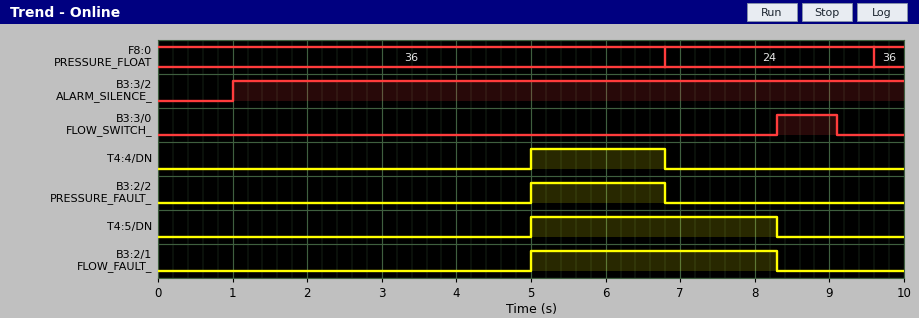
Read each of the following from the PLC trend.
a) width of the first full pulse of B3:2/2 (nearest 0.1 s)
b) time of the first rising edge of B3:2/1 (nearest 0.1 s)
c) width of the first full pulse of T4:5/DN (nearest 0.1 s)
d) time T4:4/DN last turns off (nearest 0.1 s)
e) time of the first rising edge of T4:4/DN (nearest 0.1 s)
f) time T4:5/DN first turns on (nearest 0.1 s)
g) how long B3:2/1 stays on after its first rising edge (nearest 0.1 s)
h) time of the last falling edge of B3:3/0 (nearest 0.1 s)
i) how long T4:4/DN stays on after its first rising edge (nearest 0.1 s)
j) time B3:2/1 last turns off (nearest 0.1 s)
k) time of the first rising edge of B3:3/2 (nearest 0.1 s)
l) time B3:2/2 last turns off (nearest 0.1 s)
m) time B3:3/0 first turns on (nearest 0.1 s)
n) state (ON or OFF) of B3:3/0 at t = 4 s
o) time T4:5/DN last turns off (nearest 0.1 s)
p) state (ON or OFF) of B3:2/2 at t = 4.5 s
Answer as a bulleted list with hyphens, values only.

- 1.8 s
- 5.0 s
- 3.3 s
- 6.8 s
- 5.0 s
- 5.0 s
- 3.3 s
- 9.1 s
- 1.8 s
- 8.3 s
- 1.0 s
- 6.8 s
- 8.3 s
- OFF
- 8.3 s
- OFF
